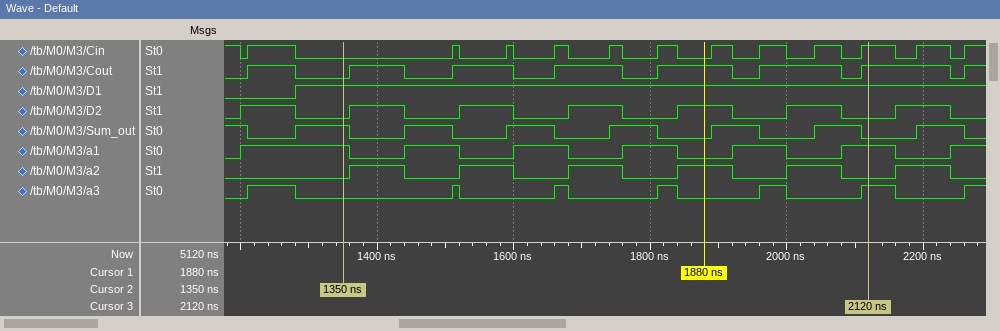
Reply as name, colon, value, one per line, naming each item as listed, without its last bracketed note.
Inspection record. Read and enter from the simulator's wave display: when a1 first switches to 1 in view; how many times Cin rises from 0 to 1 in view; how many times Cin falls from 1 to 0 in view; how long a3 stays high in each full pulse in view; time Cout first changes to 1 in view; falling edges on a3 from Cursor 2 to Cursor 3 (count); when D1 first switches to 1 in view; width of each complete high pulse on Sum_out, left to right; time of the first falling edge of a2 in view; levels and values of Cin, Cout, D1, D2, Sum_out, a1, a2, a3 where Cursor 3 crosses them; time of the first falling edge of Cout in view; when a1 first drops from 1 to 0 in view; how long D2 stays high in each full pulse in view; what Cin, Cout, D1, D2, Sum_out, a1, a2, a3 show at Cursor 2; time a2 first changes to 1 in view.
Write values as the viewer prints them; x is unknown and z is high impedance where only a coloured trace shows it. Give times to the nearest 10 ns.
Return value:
when a1 first switches to 1 in view: 1200 ns
how many times Cin rises from 0 to 1 in view: 12
how many times Cin falls from 1 to 0 in view: 12
how long a3 stays high in each full pulse in view: 70 ns, 10 ns, 20 ns, 30 ns, 40 ns, 50 ns
time Cout first changes to 1 in view: 1210 ns
falling edges on a3 from Cursor 2 to Cursor 3: 4
when D1 first switches to 1 in view: 1280 ns
width of each complete high pulse on Sum_out, left to right: 80 ns, 70 ns, 70 ns, 70 ns, 70 ns, 70 ns, 70 ns
time of the first falling edge of a2 in view: 1440 ns
levels and values of Cin, Cout, D1, D2, Sum_out, a1, a2, a3 where Cursor 3 crosses them: Cin=1, Cout=1, D1=1, D2=0, Sum_out=0, a1=1, a2=0, a3=1
time of the first falling edge of Cout in view: 1280 ns
when a1 first drops from 1 to 0 in view: 1360 ns
how long D2 stays high in each full pulse in view: 80 ns, 80 ns, 80 ns, 80 ns, 80 ns, 80 ns, 80 ns
what Cin, Cout, D1, D2, Sum_out, a1, a2, a3 show at Cursor 2: Cin=0, Cout=0, D1=1, D2=0, Sum_out=1, a1=1, a2=0, a3=0
time a2 first changes to 1 in view: 1360 ns
